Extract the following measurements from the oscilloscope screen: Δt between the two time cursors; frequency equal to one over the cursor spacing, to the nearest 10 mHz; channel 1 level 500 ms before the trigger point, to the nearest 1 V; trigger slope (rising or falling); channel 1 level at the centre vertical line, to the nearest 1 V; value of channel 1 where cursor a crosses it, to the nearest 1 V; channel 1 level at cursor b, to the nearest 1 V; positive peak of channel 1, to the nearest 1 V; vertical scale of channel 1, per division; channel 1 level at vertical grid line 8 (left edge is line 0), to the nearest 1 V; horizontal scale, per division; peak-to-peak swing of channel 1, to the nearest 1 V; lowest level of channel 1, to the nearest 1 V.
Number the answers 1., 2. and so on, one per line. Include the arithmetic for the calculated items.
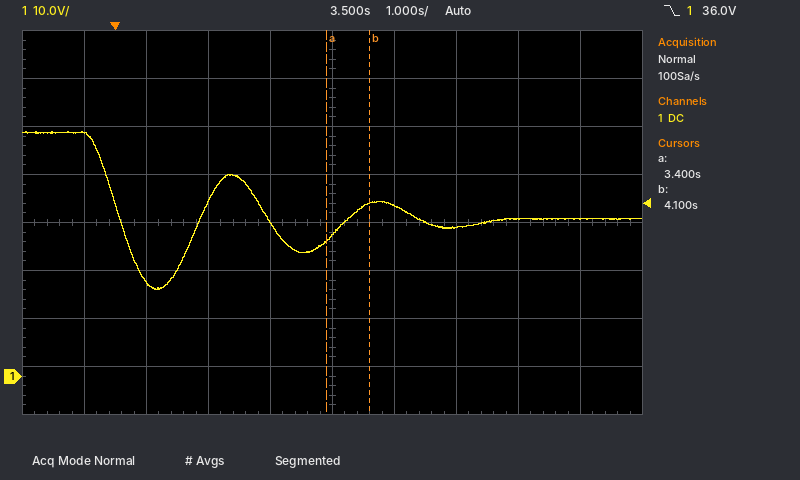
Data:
1. 4.1 s − (3.4 s) = 700 ms
2. 1 / 700 ms ≈ 1.43 Hz
3. 51 V
4. falling
5. 29 V
6. 28 V
7. 36 V
8. 51 V
9. 10 V
10. 33 V
11. 1 s
12. 51 V − (18 V) = 33 V
13. 18 V
